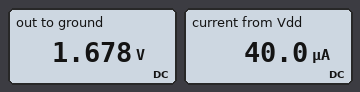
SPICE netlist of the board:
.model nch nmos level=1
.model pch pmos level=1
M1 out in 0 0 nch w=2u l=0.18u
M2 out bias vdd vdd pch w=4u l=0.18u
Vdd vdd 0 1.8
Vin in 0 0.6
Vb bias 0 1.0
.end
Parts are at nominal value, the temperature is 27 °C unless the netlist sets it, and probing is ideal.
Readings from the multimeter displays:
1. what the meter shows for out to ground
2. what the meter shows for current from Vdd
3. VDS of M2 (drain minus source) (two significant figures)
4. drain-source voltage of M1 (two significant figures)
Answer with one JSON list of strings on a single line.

["1.678 V", "40.0 µA", "-120 mV", "1.7 V"]
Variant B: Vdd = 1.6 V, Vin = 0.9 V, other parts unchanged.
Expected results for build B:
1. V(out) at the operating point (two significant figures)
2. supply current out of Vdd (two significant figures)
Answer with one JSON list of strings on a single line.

["600 mV", "80 µA"]
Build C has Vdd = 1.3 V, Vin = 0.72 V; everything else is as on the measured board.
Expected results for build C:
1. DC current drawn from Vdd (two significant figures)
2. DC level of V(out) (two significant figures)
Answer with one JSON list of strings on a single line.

["20 µA", "140 mV"]
